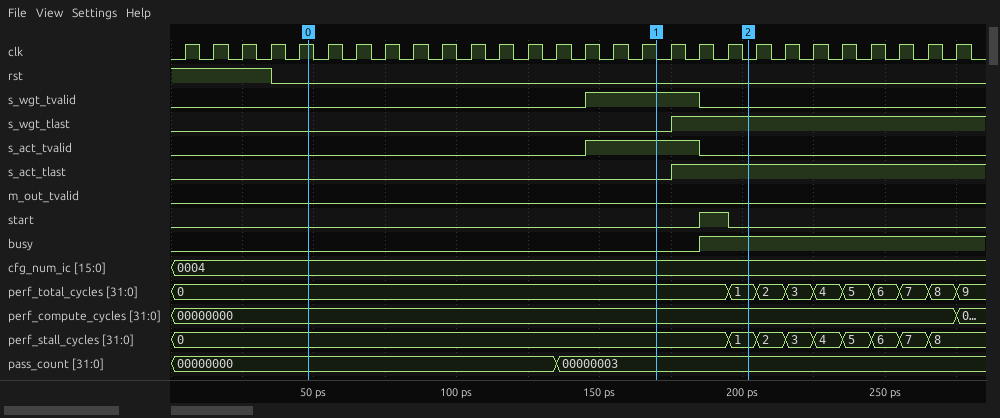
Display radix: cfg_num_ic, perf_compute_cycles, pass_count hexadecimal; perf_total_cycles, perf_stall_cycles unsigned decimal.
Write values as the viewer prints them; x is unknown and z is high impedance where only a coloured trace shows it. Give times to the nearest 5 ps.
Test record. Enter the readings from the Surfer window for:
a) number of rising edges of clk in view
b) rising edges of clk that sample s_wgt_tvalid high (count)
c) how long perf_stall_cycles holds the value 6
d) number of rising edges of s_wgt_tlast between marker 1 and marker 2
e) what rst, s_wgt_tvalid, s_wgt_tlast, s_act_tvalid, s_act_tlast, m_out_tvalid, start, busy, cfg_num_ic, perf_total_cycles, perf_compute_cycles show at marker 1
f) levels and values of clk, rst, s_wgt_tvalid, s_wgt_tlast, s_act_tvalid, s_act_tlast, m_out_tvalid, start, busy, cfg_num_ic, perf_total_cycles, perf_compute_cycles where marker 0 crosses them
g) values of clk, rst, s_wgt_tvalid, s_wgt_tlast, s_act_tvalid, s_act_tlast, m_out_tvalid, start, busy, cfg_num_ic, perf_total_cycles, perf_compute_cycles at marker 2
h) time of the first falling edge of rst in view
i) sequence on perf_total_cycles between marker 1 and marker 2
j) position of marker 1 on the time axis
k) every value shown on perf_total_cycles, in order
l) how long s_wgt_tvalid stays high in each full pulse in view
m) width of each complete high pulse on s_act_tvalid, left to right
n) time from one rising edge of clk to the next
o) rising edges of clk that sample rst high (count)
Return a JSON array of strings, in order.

["28", "4", "10 ps", "1", "rst=0, s_wgt_tvalid=1, s_wgt_tlast=0, s_act_tvalid=1, s_act_tlast=0, m_out_tvalid=0, start=0, busy=0, cfg_num_ic=0004, perf_total_cycles=0, perf_compute_cycles=00000000", "clk=1, rst=0, s_wgt_tvalid=0, s_wgt_tlast=0, s_act_tvalid=0, s_act_tlast=0, m_out_tvalid=0, start=0, busy=0, cfg_num_ic=0004, perf_total_cycles=0, perf_compute_cycles=00000000", "clk=0, rst=0, s_wgt_tvalid=0, s_wgt_tlast=1, s_act_tvalid=0, s_act_tlast=1, m_out_tvalid=0, start=0, busy=1, cfg_num_ic=0004, perf_total_cycles=1, perf_compute_cycles=00000000", "35 ps", "0, 1", "170 ps", "0, 1, 2, 3, 4, 5, 6, 7, 8, 9", "40 ps", "40 ps", "10 ps", "4"]
